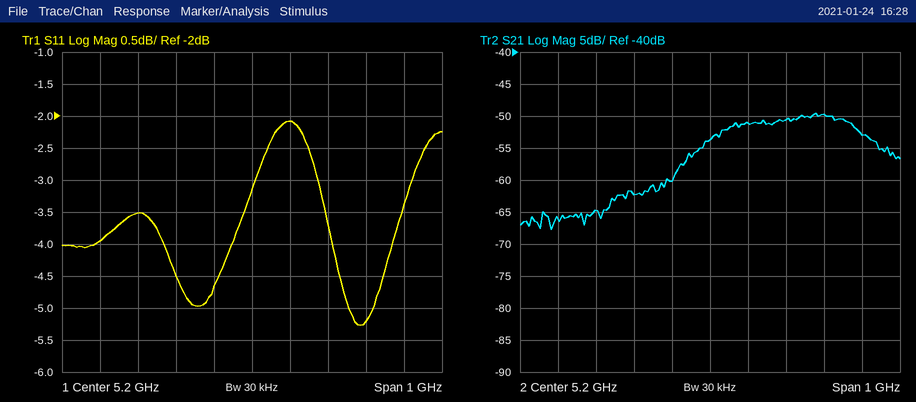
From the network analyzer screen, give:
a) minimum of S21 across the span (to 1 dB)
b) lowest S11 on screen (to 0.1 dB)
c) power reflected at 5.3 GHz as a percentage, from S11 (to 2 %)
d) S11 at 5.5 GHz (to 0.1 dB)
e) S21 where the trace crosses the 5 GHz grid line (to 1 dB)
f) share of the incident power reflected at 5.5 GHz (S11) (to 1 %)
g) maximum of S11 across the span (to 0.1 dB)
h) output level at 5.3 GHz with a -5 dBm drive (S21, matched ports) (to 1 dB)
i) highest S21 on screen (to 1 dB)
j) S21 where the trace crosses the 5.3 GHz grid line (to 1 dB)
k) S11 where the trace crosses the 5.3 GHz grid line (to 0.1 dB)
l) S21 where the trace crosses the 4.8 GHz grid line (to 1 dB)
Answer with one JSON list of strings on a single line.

["-68 dB", "-5.3 dB", "62 %", "-5.2 dB", "-62 dB", "30 %", "-2.1 dB", "-56 dBm", "-50 dB", "-51 dB", "-2.1 dB", "-66 dB"]
